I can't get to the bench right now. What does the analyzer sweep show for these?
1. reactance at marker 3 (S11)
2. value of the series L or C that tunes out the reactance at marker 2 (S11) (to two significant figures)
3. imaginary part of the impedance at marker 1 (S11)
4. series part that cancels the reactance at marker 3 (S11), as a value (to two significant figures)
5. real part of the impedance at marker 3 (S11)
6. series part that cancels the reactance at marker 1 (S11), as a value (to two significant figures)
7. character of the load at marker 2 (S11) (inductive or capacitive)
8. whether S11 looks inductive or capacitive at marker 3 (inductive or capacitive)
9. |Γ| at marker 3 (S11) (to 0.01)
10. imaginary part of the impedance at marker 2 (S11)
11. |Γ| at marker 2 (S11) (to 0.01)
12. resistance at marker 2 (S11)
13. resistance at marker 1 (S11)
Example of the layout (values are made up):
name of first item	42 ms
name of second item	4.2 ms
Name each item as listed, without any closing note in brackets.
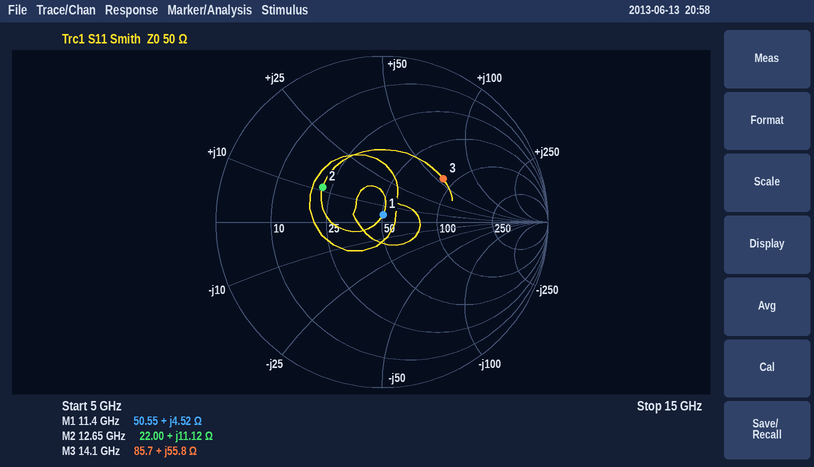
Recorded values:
reactance at marker 3	+55.8 Ω
value of the series L or C that tunes out the reactance at marker 2 (S11)	1.1 pF
imaginary part of the impedance at marker 1	+4.52 Ω
series part that cancels the reactance at marker 3 (S11), as a value	200 fF
real part of the impedance at marker 3	85.7 Ω
series part that cancels the reactance at marker 1 (S11), as a value	3.1 pF
character of the load at marker 2 (S11)	inductive
whether S11 looks inductive or capacitive at marker 3	inductive
|Γ| at marker 3 (S11)	0.45
imaginary part of the impedance at marker 2	+11.12 Ω
|Γ| at marker 2 (S11)	0.41
resistance at marker 2	22.00 Ω
resistance at marker 1	50.55 Ω
